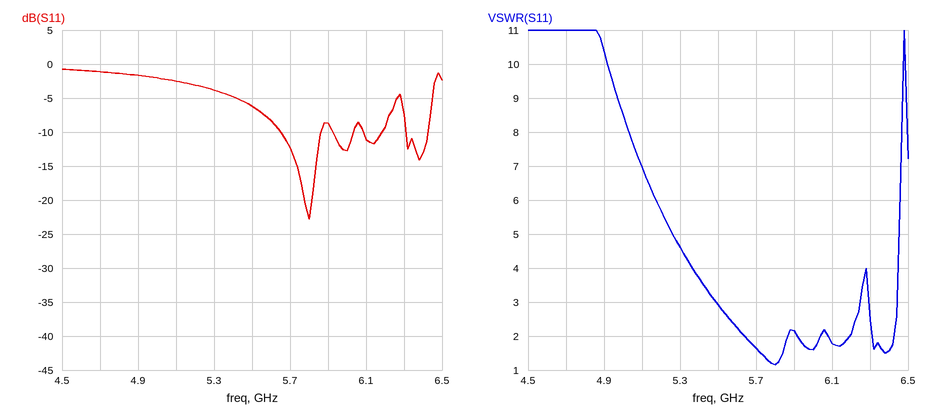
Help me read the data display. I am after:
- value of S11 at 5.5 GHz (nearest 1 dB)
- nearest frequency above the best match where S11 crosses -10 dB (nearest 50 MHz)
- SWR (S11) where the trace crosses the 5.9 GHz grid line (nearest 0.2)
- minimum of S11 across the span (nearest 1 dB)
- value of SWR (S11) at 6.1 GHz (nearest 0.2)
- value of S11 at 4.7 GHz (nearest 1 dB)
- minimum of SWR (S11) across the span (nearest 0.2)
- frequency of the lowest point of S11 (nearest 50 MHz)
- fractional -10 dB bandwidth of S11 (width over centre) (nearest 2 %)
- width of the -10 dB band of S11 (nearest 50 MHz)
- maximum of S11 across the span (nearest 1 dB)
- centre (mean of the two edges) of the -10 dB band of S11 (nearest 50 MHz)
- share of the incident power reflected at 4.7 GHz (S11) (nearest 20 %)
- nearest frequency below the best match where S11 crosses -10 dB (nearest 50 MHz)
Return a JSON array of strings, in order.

["-6 dB", "5.85 GHz", "2.2", "-23 dB", "1.8", "-1 dB", "1.2", "5.80 GHz", "4 %", "200 MHz", "-1 dB", "5.75 GHz", "80 %", "5.65 GHz"]
